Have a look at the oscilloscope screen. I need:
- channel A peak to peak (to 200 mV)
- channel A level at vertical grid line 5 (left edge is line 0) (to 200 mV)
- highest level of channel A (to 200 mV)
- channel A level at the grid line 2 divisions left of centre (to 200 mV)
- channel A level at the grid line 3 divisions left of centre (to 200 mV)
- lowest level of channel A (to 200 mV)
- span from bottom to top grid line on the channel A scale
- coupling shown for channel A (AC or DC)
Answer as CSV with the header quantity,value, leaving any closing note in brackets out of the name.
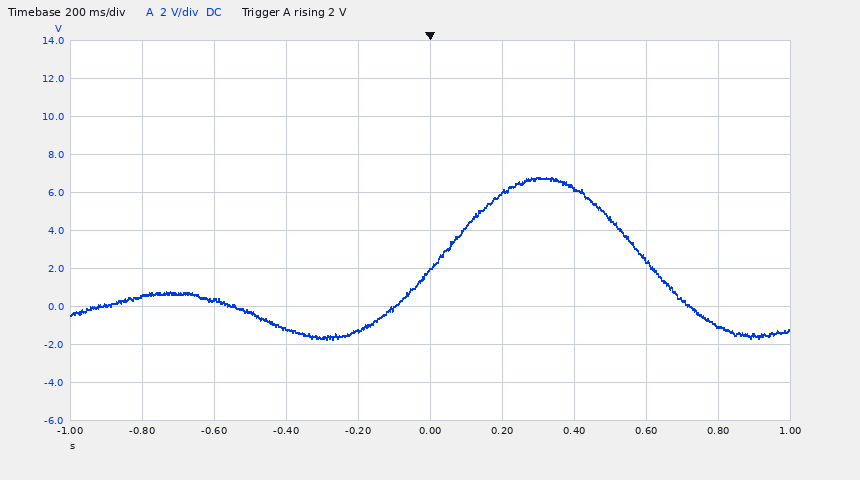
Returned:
quantity,value
channel A peak to peak,8.6 V
channel A level at vertical grid line 5 (left edge is line 0),2.0 V
highest level of channel A,6.8 V
channel A level at the grid line 2 divisions left of centre,-1.2 V
channel A level at the grid line 3 divisions left of centre,400 mV
lowest level of channel A,-1.8 V
span from bottom to top grid line on the channel A scale,20 V
coupling shown for channel A,DC
